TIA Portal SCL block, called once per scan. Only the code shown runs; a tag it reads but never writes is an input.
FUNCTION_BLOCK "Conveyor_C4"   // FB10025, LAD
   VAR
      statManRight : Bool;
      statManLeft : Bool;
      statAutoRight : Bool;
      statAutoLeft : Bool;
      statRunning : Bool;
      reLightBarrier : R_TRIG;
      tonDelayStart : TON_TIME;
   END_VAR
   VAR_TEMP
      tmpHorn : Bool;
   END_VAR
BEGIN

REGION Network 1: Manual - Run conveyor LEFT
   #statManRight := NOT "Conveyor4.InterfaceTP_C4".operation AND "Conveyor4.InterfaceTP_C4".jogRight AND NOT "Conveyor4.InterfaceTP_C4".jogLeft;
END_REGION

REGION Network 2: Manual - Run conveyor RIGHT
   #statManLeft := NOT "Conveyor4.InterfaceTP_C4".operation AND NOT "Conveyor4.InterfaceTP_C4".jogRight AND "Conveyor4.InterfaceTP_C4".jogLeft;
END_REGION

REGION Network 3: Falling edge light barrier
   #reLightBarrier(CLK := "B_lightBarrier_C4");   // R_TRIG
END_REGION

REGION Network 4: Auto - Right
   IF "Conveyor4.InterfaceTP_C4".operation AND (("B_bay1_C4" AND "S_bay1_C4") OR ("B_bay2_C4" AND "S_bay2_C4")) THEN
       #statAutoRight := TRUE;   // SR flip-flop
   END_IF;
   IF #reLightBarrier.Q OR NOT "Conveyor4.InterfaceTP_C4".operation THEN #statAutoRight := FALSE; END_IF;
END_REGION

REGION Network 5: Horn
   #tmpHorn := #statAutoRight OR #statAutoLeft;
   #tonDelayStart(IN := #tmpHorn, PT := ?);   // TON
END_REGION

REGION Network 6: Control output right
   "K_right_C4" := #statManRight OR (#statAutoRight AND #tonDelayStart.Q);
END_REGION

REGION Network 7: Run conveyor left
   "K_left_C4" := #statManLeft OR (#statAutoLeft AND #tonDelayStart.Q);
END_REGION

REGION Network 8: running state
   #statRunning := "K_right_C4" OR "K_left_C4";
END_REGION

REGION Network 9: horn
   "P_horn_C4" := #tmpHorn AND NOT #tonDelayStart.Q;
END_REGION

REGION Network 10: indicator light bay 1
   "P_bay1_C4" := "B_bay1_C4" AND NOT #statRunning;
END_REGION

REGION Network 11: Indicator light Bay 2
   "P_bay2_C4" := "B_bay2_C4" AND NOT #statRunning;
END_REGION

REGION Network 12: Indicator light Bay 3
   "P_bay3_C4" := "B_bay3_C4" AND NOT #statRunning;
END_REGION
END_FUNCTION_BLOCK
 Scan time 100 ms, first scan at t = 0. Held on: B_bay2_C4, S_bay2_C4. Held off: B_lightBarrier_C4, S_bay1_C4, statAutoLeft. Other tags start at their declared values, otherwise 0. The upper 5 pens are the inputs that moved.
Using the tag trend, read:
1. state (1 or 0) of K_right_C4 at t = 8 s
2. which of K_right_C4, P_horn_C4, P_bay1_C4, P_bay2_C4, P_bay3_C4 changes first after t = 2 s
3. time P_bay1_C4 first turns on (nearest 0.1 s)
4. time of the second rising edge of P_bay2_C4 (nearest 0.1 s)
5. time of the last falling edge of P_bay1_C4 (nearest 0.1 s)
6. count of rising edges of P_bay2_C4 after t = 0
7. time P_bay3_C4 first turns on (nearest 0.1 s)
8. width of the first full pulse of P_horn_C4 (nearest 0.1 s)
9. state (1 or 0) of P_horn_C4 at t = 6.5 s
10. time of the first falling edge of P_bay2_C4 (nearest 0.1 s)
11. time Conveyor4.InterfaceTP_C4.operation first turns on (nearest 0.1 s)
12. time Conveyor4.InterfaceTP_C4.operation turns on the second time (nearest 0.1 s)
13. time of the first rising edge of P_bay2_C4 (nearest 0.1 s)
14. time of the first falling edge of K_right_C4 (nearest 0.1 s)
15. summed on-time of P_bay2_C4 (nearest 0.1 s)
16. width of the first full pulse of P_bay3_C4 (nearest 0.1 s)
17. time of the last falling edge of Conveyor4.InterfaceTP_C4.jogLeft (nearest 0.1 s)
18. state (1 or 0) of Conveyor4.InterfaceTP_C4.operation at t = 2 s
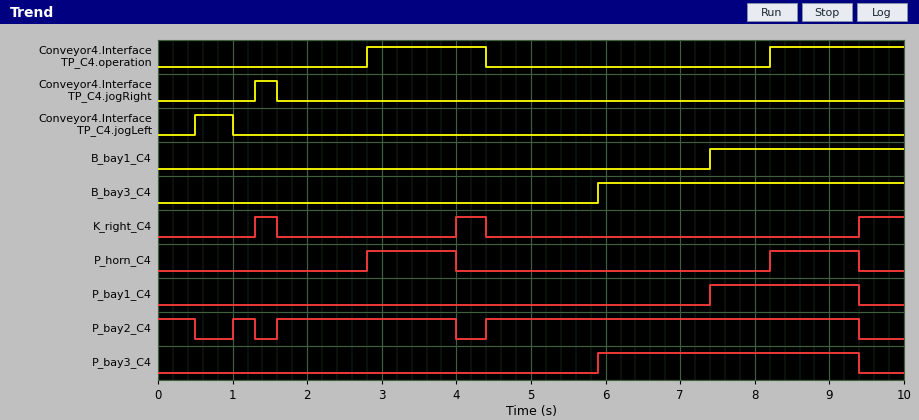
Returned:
0
P_horn_C4
7.4 s
1.6 s
9.4 s
3
5.9 s
1.2 s
0
0.5 s
2.8 s
8.2 s
1.0 s
1.6 s
8.2 s
3.5 s
1.0 s
0
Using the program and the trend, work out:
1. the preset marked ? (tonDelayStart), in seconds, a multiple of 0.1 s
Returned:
1.2 s
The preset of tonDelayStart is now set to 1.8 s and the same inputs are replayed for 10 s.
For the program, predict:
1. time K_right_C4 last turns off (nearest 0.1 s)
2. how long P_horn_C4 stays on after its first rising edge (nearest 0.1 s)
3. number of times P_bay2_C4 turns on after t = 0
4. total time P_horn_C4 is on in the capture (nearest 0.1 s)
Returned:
1.6 s
1.6 s
2
3.4 s
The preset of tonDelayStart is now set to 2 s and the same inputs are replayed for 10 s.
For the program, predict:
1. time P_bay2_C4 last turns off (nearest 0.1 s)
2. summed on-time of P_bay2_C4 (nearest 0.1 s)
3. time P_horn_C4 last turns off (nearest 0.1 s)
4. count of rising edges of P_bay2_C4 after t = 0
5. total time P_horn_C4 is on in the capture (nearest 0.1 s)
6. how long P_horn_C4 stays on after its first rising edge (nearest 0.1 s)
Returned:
1.3 s
9.2 s
4.4 s
2
3.4 s
1.6 s
